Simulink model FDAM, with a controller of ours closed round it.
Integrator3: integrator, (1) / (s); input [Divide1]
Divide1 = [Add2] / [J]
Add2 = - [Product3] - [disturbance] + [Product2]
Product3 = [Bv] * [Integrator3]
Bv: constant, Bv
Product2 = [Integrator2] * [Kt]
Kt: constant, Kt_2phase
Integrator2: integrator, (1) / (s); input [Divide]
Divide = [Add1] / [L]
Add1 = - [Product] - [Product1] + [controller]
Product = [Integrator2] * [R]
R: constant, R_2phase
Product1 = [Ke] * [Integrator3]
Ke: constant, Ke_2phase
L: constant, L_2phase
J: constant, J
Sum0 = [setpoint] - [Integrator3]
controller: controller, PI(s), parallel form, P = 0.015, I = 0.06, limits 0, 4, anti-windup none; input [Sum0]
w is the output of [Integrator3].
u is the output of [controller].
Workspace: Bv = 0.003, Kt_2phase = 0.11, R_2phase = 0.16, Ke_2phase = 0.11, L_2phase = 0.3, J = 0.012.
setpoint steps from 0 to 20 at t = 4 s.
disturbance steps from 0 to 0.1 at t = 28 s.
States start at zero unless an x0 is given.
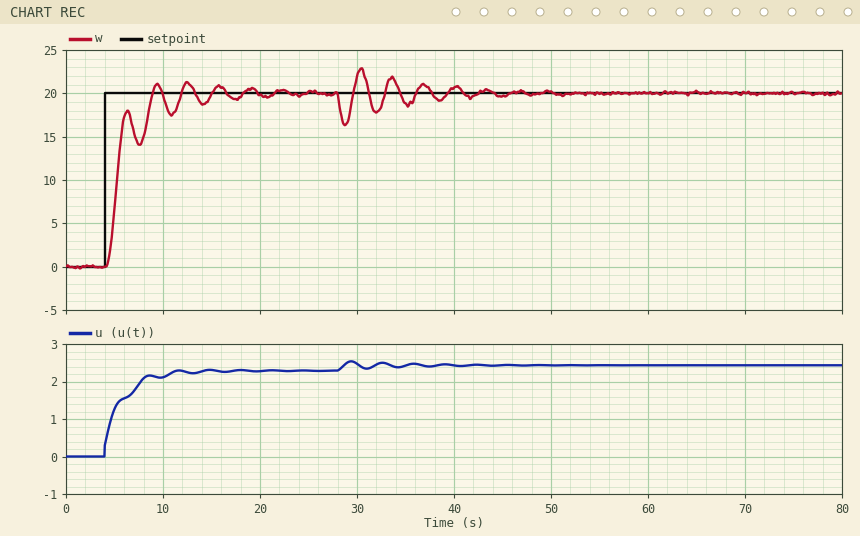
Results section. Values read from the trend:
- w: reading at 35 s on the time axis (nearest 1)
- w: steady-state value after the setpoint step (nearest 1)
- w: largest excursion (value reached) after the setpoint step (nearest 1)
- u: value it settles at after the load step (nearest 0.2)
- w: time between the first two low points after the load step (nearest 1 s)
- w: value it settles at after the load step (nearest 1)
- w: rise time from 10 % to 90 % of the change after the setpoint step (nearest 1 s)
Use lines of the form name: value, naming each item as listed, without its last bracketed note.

w: reading at 35 s on the time axis: 19
w: steady-state value after the setpoint step: 20
w: largest excursion (value reached) after the setpoint step: 21
u: value it settles at after the load step: 2.4
w: time between the first two low points after the load step: 3 s
w: value it settles at after the load step: 20
w: rise time from 10 % to 90 % of the change after the setpoint step: 4 s
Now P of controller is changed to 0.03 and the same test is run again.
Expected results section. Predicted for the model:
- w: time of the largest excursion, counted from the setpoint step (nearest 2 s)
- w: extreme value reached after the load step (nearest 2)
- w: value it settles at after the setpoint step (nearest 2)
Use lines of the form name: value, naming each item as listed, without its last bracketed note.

w: time of the largest excursion, counted from the setpoint step: 8 s
w: extreme value reached after the load step: 16
w: value it settles at after the setpoint step: 20
